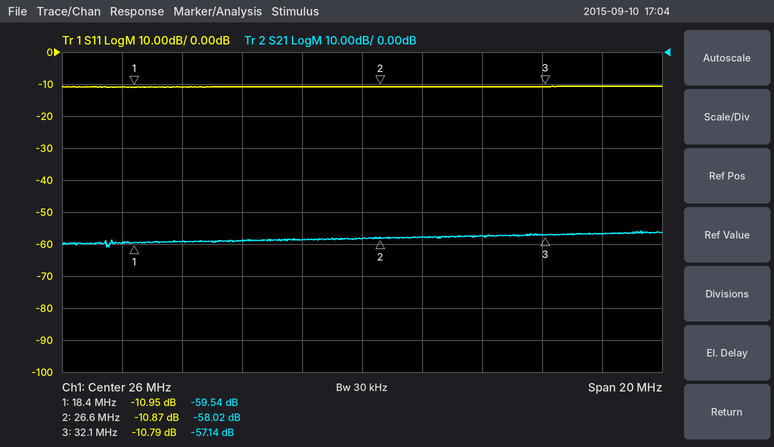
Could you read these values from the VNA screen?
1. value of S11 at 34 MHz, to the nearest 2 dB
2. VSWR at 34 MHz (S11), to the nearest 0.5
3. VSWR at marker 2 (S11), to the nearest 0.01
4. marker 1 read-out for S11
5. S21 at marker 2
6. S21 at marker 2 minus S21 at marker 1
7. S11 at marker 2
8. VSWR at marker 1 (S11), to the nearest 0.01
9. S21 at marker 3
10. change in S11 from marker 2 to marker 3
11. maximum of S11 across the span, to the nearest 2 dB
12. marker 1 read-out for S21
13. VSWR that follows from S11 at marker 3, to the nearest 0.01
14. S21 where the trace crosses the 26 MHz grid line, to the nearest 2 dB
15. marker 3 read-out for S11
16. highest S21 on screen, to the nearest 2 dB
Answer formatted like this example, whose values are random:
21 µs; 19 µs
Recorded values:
-10 dB; 2.0; 1.80; -10.95 dB; -58.02 dB; 1.52 dB; -10.87 dB; 1.79; -57.14 dB; 0.08 dB; -10 dB; -59.54 dB; 1.81; -58 dB; -10.79 dB; -56 dB
